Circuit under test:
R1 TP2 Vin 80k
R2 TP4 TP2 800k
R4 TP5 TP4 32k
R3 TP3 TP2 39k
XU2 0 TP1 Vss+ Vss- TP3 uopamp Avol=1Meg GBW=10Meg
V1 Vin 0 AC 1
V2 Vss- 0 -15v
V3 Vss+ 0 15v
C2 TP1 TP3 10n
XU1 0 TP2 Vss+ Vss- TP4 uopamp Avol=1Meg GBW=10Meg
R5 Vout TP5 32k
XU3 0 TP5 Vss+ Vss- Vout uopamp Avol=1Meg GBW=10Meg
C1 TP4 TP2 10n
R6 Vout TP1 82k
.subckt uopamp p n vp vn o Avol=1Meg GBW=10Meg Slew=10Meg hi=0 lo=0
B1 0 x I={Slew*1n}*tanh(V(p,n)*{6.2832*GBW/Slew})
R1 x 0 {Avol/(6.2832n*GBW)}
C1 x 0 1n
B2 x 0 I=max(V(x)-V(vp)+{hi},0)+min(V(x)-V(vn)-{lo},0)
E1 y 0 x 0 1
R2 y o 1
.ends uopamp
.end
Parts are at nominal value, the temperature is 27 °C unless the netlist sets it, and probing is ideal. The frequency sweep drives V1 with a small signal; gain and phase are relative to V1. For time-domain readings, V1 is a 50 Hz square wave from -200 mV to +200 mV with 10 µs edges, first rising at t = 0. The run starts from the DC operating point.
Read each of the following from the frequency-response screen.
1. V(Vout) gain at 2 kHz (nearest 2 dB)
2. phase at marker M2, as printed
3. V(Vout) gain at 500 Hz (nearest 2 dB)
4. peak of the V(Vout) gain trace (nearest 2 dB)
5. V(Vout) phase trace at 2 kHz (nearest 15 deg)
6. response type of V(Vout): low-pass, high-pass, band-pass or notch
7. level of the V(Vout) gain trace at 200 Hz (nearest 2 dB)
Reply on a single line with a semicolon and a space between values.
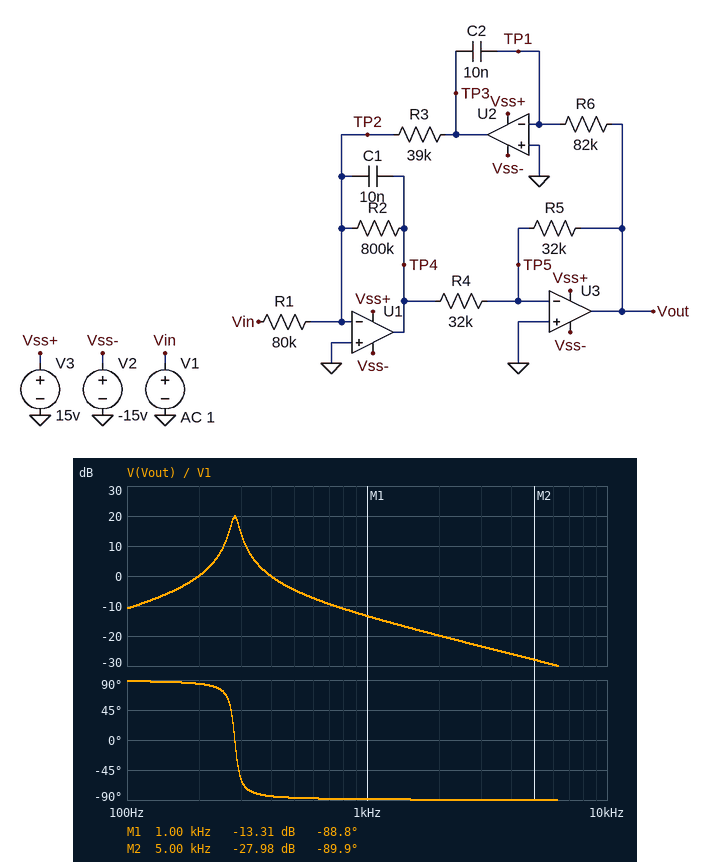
-20 dB; -89.9 deg; -4 dB; 20 dB; -90 deg; band-pass; 0 dB
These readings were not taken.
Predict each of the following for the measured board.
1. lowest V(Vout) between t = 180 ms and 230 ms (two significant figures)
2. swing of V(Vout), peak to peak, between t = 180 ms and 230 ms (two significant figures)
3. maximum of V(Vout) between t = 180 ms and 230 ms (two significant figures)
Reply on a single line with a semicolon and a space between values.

-210 mV; 420 mV; 210 mV
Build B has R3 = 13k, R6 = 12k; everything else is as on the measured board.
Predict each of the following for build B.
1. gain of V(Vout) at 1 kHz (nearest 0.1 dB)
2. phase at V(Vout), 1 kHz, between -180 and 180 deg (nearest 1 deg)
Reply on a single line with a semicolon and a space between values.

-9.9 dB; 88 deg
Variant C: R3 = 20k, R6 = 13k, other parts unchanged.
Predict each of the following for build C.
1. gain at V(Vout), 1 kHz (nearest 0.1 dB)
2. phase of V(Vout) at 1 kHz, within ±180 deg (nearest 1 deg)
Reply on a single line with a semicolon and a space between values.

15.7 dB; -53 deg
